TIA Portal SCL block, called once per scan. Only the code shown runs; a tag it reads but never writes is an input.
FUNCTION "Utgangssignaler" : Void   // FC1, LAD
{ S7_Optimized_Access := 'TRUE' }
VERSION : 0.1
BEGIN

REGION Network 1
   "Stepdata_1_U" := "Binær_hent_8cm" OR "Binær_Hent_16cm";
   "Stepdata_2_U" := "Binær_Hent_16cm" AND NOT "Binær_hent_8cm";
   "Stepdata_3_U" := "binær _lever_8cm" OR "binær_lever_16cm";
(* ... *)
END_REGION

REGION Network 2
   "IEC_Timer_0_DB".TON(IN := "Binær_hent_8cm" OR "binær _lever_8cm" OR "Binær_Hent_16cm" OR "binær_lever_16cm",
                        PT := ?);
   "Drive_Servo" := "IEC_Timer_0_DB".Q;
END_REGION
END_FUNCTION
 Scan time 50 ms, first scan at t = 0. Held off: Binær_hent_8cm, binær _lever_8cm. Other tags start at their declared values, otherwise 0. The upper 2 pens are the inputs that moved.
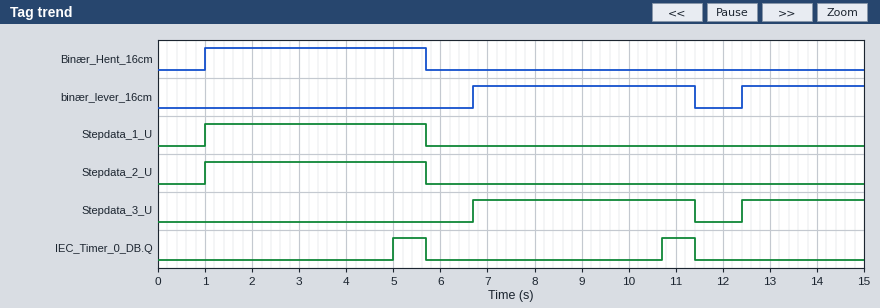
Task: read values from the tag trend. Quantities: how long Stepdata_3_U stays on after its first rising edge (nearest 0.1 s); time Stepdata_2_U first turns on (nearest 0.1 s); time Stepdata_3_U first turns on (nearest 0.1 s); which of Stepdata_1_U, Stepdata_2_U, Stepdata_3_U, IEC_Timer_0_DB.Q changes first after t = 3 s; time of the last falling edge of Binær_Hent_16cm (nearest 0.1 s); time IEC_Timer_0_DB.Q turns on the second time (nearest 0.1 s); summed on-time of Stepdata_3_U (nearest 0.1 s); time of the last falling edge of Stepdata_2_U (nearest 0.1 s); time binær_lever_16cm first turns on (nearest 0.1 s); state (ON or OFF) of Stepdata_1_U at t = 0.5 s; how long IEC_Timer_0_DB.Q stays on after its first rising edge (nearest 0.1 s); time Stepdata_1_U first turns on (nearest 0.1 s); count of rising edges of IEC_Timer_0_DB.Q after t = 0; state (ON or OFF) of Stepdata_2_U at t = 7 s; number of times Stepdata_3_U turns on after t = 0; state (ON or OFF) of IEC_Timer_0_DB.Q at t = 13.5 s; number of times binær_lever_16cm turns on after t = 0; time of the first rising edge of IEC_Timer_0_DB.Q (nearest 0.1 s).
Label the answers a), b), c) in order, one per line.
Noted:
a) 4.7 s
b) 1.0 s
c) 6.7 s
d) IEC_Timer_0_DB.Q
e) 5.7 s
f) 10.7 s
g) 7.3 s
h) 5.7 s
i) 6.7 s
j) OFF
k) 0.7 s
l) 1.0 s
m) 2
n) OFF
o) 2
p) OFF
q) 2
r) 5.0 s
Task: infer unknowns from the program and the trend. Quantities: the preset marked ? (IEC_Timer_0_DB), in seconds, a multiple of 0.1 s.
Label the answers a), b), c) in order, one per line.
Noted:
a) 4.0 s
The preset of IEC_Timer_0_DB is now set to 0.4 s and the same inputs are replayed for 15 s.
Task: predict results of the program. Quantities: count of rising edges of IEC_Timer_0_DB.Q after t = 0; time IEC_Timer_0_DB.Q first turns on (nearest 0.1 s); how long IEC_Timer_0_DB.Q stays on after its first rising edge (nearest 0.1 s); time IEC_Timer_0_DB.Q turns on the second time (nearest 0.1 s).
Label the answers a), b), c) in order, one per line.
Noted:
a) 3
b) 1.4 s
c) 4.3 s
d) 7.1 s
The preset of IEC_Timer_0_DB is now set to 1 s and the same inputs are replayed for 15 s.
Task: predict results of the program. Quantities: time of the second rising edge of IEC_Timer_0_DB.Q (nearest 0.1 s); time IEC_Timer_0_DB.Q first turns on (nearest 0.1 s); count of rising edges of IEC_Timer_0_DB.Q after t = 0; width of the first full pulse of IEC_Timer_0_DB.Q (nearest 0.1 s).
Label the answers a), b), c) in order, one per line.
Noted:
a) 7.7 s
b) 2.0 s
c) 3
d) 3.7 s
